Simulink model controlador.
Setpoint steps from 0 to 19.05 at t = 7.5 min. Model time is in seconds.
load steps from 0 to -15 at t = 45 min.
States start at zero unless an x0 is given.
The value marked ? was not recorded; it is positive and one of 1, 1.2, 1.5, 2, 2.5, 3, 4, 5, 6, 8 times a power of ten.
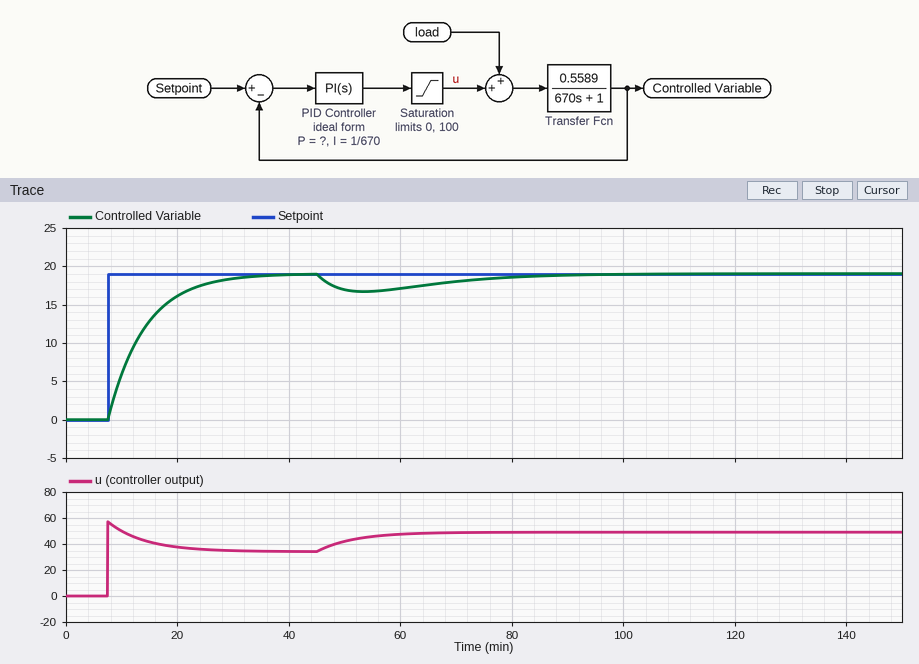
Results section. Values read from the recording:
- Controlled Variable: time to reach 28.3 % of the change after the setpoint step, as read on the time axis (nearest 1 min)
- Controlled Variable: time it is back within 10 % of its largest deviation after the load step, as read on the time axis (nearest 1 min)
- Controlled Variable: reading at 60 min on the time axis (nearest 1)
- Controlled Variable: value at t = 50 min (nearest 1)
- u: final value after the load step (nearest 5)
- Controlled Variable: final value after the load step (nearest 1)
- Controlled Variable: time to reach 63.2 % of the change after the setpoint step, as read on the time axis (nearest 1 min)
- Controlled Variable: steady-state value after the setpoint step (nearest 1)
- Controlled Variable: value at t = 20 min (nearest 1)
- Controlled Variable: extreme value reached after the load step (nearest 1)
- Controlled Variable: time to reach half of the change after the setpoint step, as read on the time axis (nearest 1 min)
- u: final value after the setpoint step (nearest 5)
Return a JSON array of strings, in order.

["10 min", "89 min", "17", "17", "50", "19", "14 min", "19", "16", "17", "12 min", "35"]
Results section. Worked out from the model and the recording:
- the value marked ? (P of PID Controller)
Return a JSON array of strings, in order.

["3"]
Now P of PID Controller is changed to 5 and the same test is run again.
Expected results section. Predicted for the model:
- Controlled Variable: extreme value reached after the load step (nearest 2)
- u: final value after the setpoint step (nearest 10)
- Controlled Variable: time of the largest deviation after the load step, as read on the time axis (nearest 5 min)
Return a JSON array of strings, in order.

["18", "30", "50 min"]
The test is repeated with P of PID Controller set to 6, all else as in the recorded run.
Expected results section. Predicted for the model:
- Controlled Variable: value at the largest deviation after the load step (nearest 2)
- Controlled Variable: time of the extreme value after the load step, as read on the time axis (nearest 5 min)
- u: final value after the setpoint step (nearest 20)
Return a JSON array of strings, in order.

["18", "50 min", "40"]
